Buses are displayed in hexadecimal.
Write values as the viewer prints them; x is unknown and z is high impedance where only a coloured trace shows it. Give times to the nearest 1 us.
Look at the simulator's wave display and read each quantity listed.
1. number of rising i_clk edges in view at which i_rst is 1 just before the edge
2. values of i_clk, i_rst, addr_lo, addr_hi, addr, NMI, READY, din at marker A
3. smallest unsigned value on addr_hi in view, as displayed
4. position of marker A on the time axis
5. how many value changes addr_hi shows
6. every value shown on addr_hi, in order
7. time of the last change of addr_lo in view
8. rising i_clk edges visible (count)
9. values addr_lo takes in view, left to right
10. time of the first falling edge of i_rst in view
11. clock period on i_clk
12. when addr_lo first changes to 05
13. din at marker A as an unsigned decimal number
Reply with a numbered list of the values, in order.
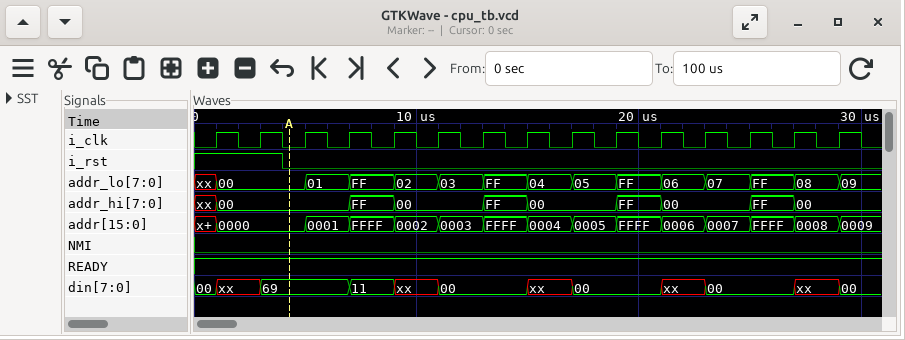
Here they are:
1. 2
2. i_clk=0, i_rst=0, addr_lo=00, addr_hi=00, addr=0000, NMI=0, READY=1, din=69
3. 00
4. 4 us
5. 9
6. xx, 00, FF, 00, FF, 00, FF, 00, FF, 00
7. 29 us
8. 15
9. xx, 00, 01, FF, 02, 03, FF, 04, 05, FF, 06, 07, FF, 08, 09
10. 4 us
11. 2 us
12. 17 us
13. 105
